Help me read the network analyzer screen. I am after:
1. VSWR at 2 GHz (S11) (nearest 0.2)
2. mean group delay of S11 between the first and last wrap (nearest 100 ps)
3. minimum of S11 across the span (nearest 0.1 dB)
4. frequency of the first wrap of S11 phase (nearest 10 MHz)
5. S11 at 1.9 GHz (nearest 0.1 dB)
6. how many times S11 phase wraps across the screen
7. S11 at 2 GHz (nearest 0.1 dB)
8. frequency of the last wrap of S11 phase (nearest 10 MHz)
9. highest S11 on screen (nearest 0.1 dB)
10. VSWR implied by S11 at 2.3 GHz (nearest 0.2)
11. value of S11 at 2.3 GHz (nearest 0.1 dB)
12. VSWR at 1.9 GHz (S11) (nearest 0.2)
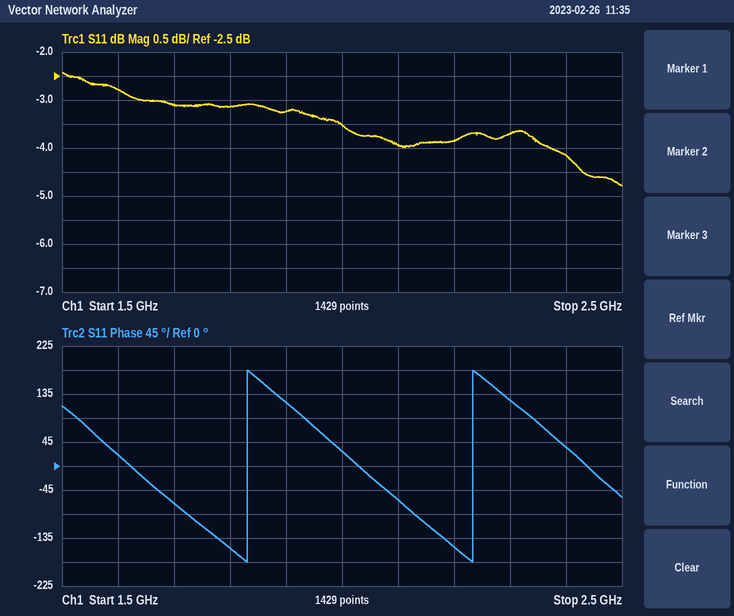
5.0
2.5 ns
-4.8 dB
1.83 GHz
-3.2 dB
2
-3.5 dB
2.23 GHz
-2.4 dB
4.8
-3.7 dB
5.4
